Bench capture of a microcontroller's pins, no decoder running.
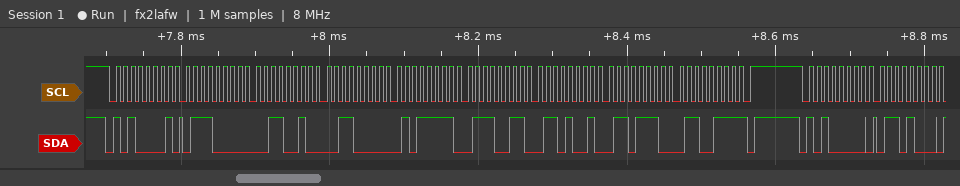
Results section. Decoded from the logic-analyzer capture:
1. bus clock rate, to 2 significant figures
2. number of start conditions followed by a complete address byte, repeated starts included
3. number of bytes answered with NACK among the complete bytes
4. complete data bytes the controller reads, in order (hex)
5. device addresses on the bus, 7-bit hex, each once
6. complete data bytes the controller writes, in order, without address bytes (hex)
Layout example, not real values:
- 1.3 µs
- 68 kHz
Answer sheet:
- 100 kHz
- 2
- 1
- 70 32 30 5F 73 69 6E 67
- 0x50
- 68
